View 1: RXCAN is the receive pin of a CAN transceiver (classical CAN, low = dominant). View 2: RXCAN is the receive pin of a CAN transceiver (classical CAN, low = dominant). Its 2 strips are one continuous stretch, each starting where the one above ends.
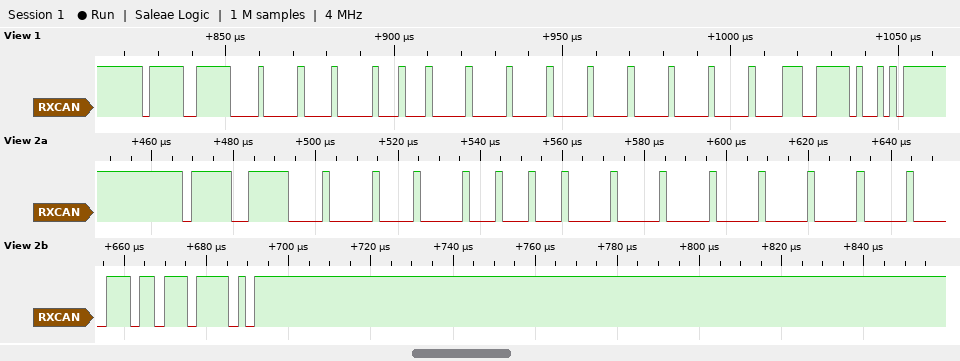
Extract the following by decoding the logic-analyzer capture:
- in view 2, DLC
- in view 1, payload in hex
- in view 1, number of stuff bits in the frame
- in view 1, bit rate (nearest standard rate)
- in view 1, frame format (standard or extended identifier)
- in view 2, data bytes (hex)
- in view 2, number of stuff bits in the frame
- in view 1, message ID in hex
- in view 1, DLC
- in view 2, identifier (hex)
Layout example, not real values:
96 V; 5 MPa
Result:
8; 02 01 10 00 00 00 00 00; 13; 500 kbit/s; standard; 02 01 11 00 00 00 00 00; 12; 0x7DF; 8; 0x7DF
